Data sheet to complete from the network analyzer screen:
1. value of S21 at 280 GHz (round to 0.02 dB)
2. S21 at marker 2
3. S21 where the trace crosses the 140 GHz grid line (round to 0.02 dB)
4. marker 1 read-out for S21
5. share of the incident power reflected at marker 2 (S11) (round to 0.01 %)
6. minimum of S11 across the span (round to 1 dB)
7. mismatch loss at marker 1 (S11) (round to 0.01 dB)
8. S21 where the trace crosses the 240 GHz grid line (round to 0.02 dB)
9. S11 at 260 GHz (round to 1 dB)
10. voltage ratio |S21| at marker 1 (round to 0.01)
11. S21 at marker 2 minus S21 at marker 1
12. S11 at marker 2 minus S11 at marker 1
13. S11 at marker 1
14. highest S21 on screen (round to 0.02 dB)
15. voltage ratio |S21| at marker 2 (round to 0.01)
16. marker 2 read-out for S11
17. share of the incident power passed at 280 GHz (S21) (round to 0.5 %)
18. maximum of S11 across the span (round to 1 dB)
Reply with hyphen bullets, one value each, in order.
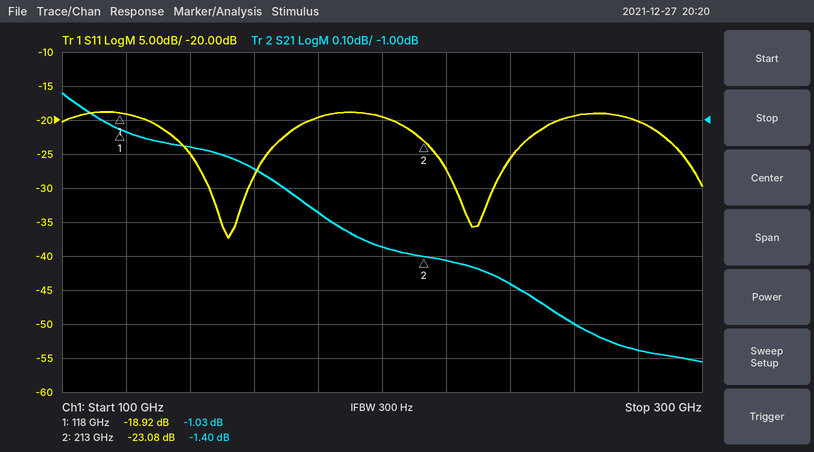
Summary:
- -1.68 dB
- -1.40 dB
- -1.08 dB
- -1.03 dB
- 0.49 %
- -37 dB
- 0.06 dB
- -1.48 dB
- -19 dB
- 0.89
- -0.37 dB
- -4.16 dB
- -18.92 dB
- -0.92 dB
- 0.85
- -23.08 dB
- 68.0 %
- -19 dB
